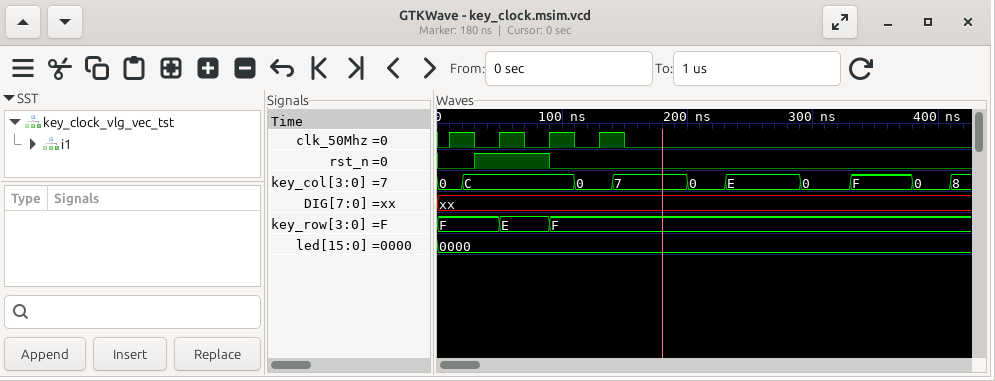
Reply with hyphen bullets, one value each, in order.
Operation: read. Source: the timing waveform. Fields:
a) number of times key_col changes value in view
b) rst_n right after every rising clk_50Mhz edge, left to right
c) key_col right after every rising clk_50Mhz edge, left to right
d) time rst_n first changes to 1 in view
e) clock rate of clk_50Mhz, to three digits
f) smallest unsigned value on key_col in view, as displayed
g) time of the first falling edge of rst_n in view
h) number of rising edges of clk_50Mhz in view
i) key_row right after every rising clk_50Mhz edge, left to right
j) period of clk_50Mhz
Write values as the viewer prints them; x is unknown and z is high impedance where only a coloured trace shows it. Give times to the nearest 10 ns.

- 9
- 0 1 0 0
- 0, C, C, 0
- 30 ns
- 25.0 MHz
- 0
- 90 ns
- 4
- F, E, F, F
- 40 ns
